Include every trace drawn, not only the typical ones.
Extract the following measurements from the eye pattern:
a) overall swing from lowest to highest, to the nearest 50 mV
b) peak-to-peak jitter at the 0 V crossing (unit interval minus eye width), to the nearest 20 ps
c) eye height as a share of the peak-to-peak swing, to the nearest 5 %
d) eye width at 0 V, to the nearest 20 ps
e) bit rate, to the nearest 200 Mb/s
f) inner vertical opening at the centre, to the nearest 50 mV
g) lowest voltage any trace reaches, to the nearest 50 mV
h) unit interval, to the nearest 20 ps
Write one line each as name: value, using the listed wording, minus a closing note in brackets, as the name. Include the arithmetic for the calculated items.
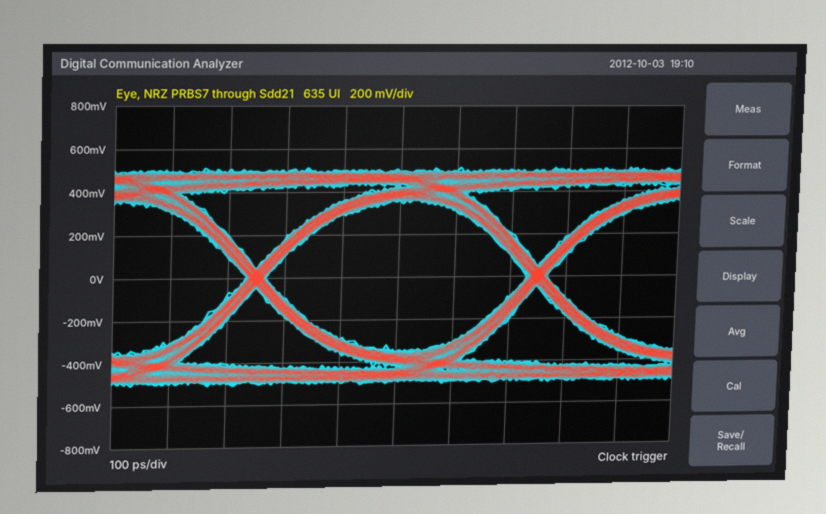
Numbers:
overall swing from lowest to highest, to the nearest 50 mV: 1.00 V
peak-to-peak jitter at the 0 V crossing (unit interval minus eye width), to the nearest 20 ps: 40 ps
eye height as a share of the peak-to-peak swing, to the nearest 5 %: 700 mV / 1.00 V ≈ 70 %
eye width at 0 V, to the nearest 20 ps: 460 ps
bit rate, to the nearest 200 Mb/s: 2.0 Gb/s
inner vertical opening at the centre, to the nearest 50 mV: 700 mV
lowest voltage any trace reaches, to the nearest 50 mV: -500 mV
unit interval, to the nearest 20 ps: 500 ps
